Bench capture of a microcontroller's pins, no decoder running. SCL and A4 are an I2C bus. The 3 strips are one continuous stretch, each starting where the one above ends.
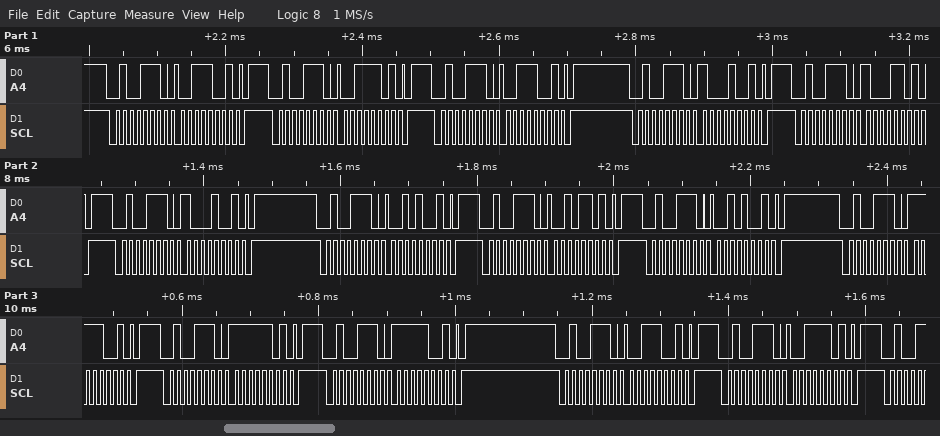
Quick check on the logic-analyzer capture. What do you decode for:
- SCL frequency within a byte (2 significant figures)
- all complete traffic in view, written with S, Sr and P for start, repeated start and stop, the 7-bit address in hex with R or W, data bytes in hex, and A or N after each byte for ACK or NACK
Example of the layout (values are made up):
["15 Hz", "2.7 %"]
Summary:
["100 kHz", "S 27W A 39 A P S 27W A 3D A P S 27W A 39 A P S 27W A 89 A P S 27W A 8D A P S 27W A 89 A P S 27W A 29 A P S 27W A 2D A P S 27W A 29 A P S 27W A F9 A P S 27W A FD A P S 27W A F9 A P S 27W A 39 A P S 27W A 3D A P"]
